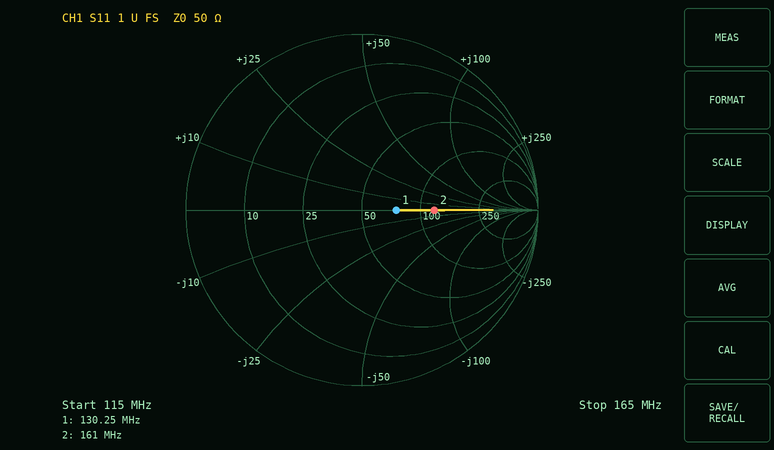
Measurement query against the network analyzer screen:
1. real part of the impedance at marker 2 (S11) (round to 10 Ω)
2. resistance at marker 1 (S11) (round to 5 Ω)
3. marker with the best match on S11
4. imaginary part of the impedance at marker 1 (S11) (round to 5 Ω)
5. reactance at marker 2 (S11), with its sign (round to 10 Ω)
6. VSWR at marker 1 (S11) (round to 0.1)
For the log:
120 Ω
75 Ω
marker 1
0 Ω
0 Ω
1.5
